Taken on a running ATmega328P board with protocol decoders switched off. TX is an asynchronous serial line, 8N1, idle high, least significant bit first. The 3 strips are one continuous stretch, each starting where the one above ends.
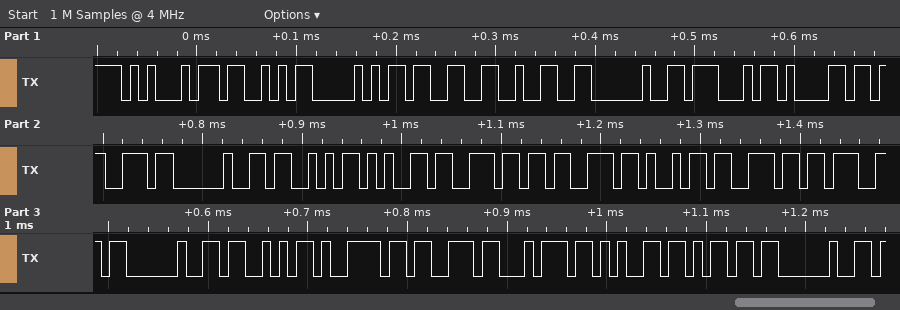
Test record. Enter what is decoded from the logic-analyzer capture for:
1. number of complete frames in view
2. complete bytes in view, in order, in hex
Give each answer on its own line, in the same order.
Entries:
25
45 53 50 33 32 20 47 61 73 20 53 65 6E 73 69 6E 67 20 53 79 73 74 65 6D 20
